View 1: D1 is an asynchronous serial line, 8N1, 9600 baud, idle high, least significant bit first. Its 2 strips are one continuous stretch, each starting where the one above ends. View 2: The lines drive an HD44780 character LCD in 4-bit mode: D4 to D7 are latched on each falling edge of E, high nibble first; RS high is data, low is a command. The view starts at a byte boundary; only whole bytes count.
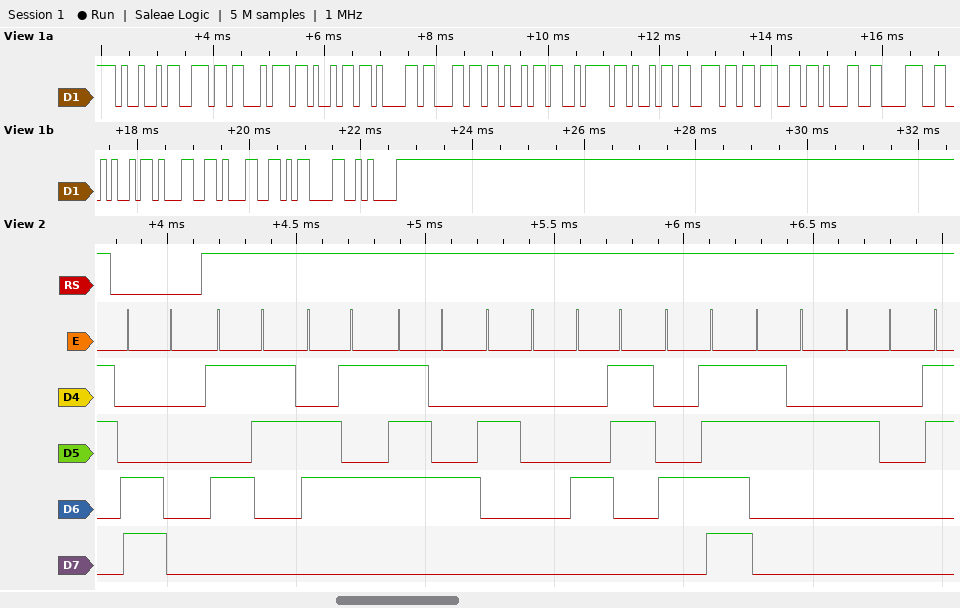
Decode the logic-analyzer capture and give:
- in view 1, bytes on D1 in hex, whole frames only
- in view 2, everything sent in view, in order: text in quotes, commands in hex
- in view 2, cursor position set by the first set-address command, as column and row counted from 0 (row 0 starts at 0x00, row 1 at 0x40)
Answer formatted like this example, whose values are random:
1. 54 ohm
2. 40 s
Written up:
1. 0x49 0x6E 0x74 0x69 0x61 0x6C 0x69 0x7A 0x69 0x6E 0x67 0x31 0x38 0x4A 0x31 0x31 0x0D 0x0A
2. 0xC0 "Set CO2 "
3. column 0, row 1
